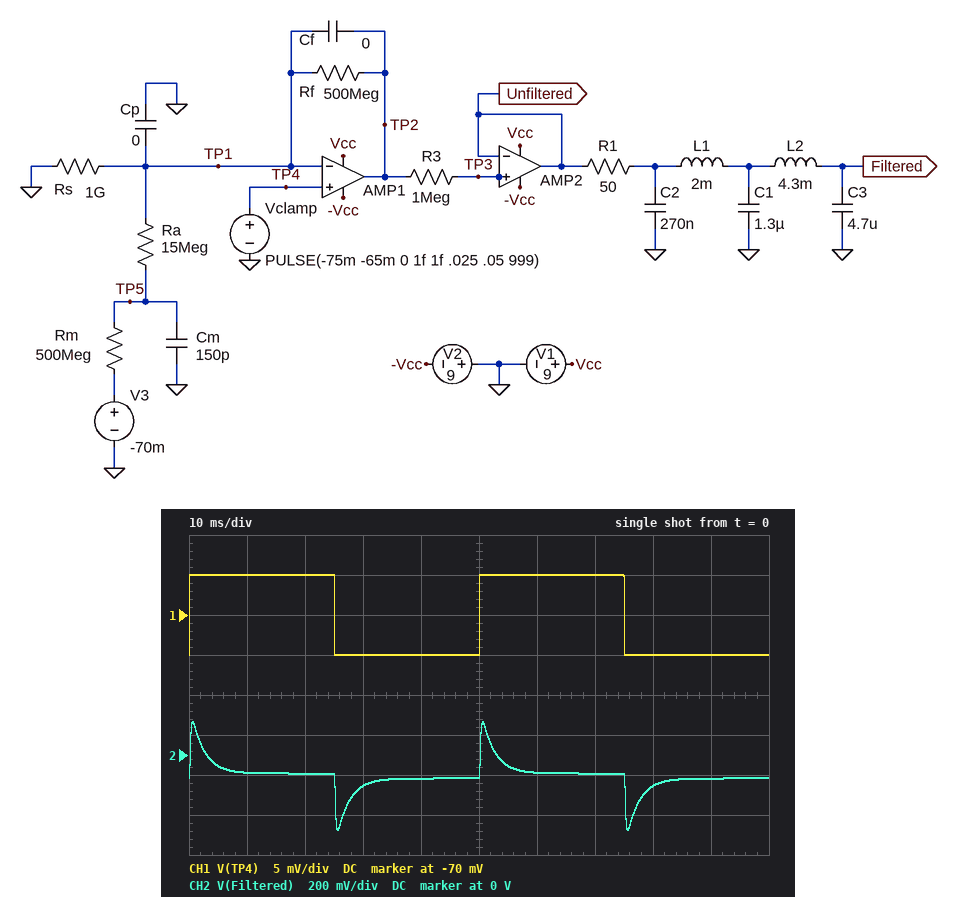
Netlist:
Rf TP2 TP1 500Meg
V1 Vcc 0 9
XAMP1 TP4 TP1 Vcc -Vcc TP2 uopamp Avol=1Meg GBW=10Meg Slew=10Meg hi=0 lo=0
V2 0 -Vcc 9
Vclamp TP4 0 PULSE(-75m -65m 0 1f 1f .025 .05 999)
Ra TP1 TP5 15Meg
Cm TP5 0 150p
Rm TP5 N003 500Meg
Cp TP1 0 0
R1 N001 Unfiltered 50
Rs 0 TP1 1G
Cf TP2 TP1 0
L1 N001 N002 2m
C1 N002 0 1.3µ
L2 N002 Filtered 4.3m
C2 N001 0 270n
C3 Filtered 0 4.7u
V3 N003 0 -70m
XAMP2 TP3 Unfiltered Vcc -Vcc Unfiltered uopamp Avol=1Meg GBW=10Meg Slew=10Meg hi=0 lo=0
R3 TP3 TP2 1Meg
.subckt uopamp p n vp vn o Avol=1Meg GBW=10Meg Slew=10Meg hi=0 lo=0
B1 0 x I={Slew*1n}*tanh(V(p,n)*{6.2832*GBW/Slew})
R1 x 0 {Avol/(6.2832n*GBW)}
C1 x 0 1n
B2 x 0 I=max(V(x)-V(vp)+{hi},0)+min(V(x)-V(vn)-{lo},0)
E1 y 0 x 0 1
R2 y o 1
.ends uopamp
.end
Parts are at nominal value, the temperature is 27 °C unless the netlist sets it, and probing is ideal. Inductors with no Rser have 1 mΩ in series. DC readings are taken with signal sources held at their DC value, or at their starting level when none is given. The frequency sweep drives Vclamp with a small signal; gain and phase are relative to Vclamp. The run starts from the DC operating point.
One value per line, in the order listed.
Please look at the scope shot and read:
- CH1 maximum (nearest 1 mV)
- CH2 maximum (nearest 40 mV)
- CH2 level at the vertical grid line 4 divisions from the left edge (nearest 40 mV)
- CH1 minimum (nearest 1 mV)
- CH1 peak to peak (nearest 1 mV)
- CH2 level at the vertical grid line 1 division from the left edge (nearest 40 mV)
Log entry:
-65 mV
160 mV
-120 mV
-75 mV
10 mV
-80 mV
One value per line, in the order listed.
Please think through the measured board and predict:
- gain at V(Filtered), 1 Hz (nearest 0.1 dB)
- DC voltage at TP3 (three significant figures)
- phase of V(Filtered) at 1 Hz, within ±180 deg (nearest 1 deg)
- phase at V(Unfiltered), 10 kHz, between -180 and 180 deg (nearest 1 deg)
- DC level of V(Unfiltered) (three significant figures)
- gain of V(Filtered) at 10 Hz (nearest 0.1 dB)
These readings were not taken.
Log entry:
8.0 dB
-117 mV
10 deg
-2 deg
-117 mV
14.5 dB
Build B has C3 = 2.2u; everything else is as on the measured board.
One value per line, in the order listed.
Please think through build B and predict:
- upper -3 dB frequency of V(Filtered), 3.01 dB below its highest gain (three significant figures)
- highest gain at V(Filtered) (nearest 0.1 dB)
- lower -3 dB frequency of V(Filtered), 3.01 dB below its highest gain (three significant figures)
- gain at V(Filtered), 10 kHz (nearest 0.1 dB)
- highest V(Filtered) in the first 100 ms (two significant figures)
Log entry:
2.34 kHz
30.6 dB
69.3 Hz
-19.9 dB
220 mV
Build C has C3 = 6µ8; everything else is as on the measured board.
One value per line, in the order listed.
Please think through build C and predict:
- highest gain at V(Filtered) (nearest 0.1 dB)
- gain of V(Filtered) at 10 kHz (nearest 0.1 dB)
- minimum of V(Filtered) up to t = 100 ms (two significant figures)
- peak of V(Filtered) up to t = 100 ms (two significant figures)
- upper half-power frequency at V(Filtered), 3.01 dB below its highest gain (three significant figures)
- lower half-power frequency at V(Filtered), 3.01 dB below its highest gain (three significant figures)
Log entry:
29.8 dB
-29.9 dB
-350 mV
140 mV
671 Hz
58.4 Hz
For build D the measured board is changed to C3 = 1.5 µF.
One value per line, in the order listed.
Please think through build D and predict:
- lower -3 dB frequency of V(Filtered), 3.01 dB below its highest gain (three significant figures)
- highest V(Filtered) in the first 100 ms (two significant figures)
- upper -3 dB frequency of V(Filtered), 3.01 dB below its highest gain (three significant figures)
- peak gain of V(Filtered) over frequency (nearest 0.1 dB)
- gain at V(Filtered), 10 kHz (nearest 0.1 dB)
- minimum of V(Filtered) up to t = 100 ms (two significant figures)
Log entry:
76.6 Hz
260 mV
3.14 kHz
31.1 dB
-16.5 dB
-470 mV
